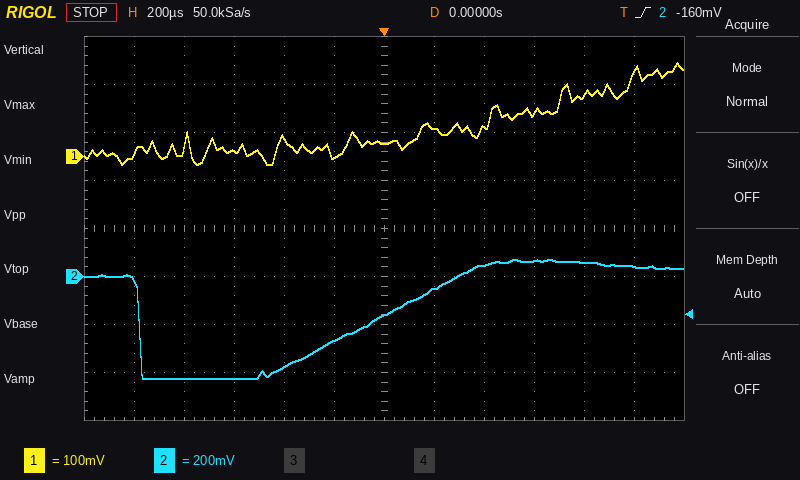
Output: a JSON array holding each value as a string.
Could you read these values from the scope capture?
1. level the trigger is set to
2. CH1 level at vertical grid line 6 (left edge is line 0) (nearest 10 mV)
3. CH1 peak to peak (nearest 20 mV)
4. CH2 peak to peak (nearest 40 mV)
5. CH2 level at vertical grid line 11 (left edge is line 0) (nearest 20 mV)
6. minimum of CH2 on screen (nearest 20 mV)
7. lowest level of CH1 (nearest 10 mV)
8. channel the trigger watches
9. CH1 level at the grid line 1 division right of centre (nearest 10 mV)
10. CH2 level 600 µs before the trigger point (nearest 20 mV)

["-160 mV", "30 mV", "220 mV", "480 mV", "40 mV", "-420 mV", "-20 mV", "CH2", "60 mV", "-420 mV"]
